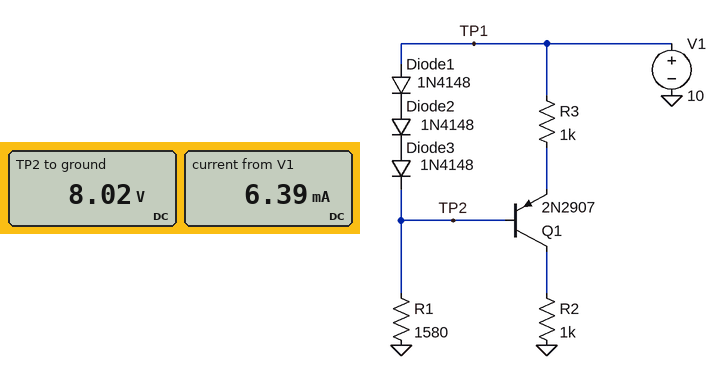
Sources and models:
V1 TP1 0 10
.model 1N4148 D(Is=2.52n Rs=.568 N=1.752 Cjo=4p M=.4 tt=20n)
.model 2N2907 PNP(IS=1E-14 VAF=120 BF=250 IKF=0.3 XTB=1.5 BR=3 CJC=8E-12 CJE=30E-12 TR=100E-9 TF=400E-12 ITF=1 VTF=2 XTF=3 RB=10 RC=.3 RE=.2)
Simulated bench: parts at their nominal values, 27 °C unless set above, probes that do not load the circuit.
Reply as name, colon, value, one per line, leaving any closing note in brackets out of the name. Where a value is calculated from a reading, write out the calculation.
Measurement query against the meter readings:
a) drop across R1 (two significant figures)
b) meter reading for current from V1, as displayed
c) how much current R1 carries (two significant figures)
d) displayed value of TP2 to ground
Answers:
drop across R1: 8.02 V = 8.0 V
meter reading for current from V1, as displayed: 6.39 mA
how much current R1 carries: (8.02 V) / 1.58 kΩ = 5.1 mA
displayed value of TP2 to ground: 8.02 V
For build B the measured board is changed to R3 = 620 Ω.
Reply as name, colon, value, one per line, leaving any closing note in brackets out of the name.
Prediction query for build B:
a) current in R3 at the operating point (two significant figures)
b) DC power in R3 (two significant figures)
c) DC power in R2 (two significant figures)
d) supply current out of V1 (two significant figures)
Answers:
current in R3 at the operating point: 2.1 mA
DC power in R3: 2.8 mW
DC power in R2: 4.4 mW
supply current out of V1: 7.2 mA
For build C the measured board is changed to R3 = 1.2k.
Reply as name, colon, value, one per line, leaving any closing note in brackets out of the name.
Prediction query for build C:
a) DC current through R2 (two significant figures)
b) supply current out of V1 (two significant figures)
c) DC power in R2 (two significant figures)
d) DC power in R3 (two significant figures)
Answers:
DC current through R2: 1.1 mA
supply current out of V1: 6.2 mA
DC power in R2: 1.2 mW
DC power in R3: 1.5 mW
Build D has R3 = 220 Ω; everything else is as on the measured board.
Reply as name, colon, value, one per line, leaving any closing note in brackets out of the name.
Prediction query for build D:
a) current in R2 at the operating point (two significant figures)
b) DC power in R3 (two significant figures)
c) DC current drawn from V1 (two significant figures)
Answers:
current in R2 at the operating point: 5.8 mA
DC power in R3: 7.4 mW
DC current drawn from V1: 11 mA
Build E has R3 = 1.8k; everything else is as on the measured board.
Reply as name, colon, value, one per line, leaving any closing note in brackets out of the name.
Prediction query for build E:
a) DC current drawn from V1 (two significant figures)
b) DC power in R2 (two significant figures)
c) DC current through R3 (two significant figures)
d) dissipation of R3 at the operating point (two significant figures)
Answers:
DC current drawn from V1: 5.8 mA
DC power in R2: 550 µW
DC current through R3: 740 µA
dissipation of R3 at the operating point: 990 µW
